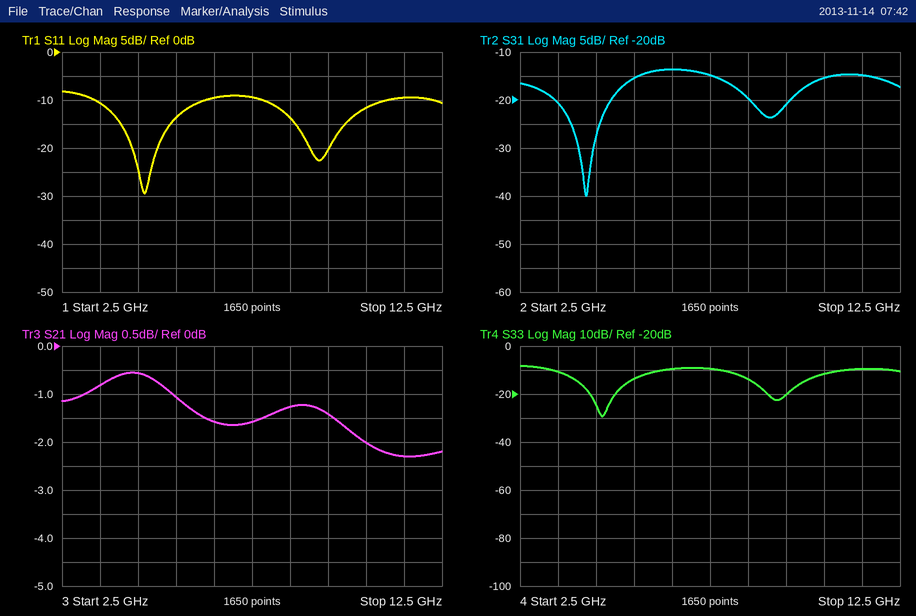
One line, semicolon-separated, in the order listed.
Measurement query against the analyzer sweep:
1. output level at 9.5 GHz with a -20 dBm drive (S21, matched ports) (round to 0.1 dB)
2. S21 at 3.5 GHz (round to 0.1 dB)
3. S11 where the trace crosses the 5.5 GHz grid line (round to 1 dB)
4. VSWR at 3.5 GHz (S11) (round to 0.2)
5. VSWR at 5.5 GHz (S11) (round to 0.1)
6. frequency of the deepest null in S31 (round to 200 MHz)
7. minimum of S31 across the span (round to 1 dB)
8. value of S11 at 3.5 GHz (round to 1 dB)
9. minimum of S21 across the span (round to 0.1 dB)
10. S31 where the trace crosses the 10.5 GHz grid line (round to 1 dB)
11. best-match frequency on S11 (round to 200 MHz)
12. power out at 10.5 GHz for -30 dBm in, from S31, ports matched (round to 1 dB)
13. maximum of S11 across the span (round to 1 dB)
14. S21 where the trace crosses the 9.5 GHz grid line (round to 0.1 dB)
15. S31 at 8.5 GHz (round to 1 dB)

-21.4 dBm; -0.8 dB; -14 dB; 1.8; 1.5; 4.2 GHz; -40 dB; -11 dB; -2.3 dB; -15 dB; 4.6 GHz; -45 dBm; -8 dB; -1.4 dB; -20 dB
